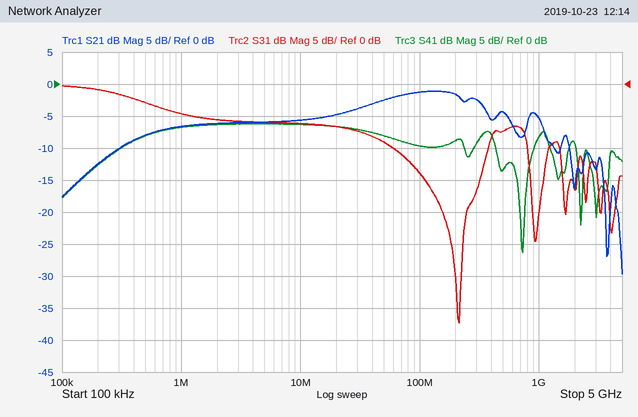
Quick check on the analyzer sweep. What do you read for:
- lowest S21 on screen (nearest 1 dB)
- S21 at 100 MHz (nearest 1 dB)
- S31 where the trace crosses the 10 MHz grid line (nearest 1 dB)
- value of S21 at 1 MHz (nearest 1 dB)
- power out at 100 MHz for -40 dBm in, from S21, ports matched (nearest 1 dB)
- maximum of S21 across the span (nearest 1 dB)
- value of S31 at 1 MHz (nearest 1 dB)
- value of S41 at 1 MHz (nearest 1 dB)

-30 dB
-1 dB
-6 dB
-7 dB
-41 dBm
-1 dB
-5 dB
-7 dB
